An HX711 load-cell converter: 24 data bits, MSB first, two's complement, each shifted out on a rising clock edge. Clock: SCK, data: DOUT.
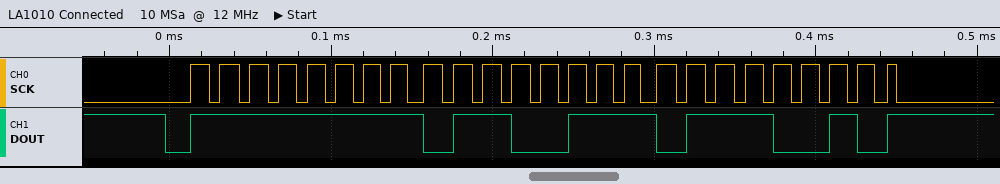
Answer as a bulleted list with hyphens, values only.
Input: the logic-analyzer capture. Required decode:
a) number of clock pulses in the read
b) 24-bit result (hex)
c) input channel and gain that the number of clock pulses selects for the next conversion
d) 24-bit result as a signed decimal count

- 25
- 0xFF6772
- channel A, gain 128
- -39054
